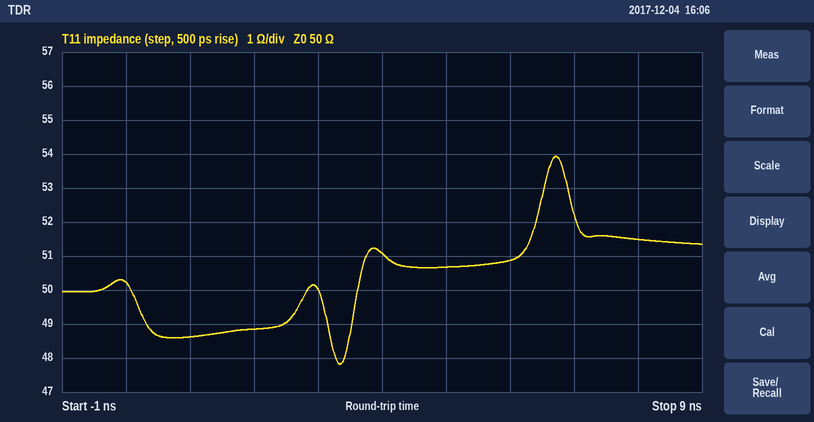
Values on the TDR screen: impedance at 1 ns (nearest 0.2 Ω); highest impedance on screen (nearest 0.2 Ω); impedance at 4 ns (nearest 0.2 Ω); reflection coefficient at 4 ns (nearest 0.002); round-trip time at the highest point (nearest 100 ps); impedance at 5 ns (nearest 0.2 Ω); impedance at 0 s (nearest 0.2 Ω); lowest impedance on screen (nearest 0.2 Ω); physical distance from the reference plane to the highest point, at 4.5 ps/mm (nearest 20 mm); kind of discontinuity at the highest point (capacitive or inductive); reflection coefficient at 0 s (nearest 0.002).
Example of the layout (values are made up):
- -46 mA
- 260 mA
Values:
- 48.6 Ω
- 54.0 Ω
- 51.0 Ω
- +0.010
- 6.7 ns
- 50.6 Ω
- 50.2 Ω
- 47.8 Ω
- 740 mm
- inductive
- +0.002
